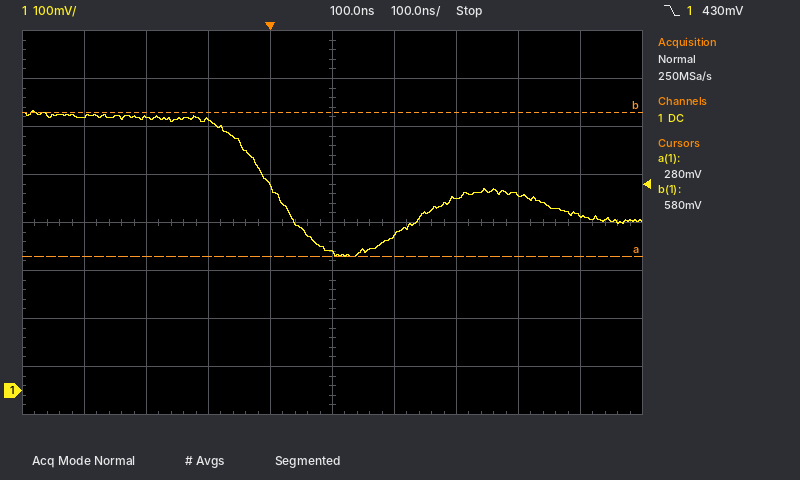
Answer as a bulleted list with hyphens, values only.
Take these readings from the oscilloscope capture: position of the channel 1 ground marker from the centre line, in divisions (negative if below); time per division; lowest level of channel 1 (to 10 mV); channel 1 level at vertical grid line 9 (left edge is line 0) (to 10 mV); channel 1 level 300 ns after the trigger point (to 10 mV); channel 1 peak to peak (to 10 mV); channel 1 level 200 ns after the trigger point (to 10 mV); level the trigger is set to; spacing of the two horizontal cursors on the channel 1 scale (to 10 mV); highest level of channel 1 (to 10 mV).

- -3.5 div
- 100 ns
- 280 mV
- 360 mV
- 400 mV
- 300 mV
- 320 mV
- 430 mV
- 300 mV
- 580 mV
